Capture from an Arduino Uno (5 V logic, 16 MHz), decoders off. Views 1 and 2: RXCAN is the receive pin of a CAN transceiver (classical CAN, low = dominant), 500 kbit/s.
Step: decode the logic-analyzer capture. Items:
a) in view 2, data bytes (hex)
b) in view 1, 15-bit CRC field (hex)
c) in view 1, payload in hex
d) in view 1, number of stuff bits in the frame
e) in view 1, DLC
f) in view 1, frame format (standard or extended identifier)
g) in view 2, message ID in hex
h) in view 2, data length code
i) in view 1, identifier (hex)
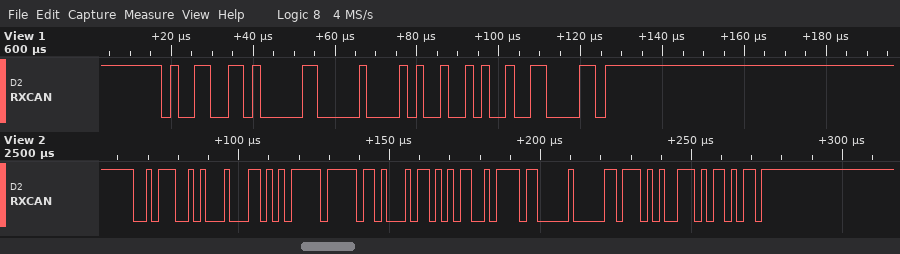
D5 FF E8 B5 65 EC 00 BA
0x5261
00 A4
2
2
standard
0x2E5
8
0x4CD
